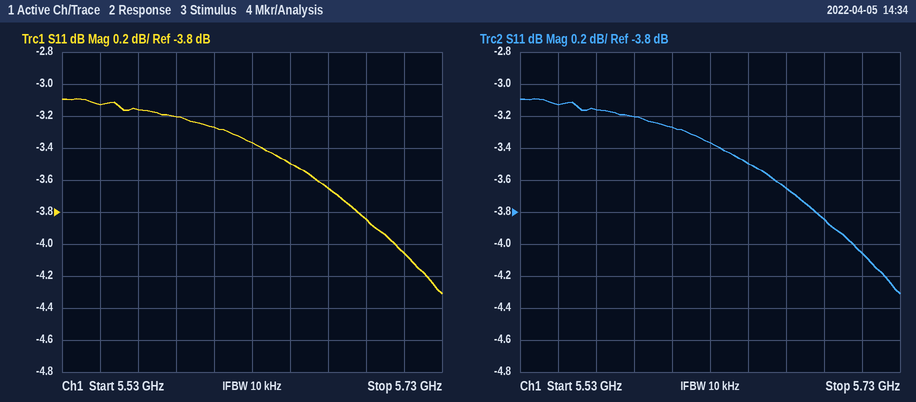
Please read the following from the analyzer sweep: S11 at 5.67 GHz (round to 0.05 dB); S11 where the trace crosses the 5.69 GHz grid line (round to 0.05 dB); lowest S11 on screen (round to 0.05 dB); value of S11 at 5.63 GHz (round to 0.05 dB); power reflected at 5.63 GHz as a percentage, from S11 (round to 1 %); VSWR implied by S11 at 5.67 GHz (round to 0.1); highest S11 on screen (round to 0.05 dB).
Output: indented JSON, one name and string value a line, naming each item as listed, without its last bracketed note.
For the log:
{
  "S11 at 5.67 GHz": "-3.65 dB",
  "S11 where the trace crosses the 5.69 GHz grid line": "-3.85 dB",
  "lowest S11 on screen": "-4.30 dB",
  "value of S11 at 5.63 GHz": "-3.35 dB",
  "power reflected at 5.63 GHz as a percentage, from S11": "46 %",
  "VSWR implied by S11 at 5.67 GHz": "4.8",
  "highest S11 on screen": "-3.10 dB"
}
